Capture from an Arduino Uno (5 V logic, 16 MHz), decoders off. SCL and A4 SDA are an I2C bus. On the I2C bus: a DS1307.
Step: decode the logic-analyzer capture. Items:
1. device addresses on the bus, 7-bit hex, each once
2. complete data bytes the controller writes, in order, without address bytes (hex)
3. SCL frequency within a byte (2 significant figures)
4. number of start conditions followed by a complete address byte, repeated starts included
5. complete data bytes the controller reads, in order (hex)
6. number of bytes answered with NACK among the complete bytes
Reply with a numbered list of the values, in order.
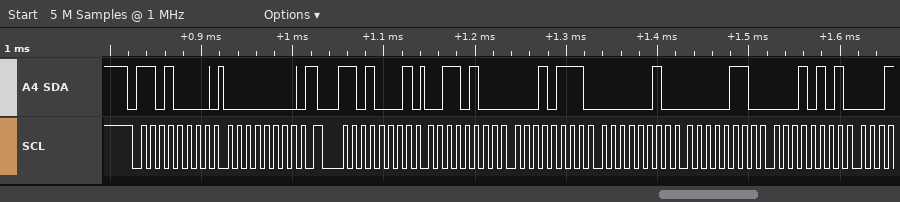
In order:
1. 0x68
2. 00
3. 100 kHz
4. 2
5. 34 17 02 06 15
6. 0
